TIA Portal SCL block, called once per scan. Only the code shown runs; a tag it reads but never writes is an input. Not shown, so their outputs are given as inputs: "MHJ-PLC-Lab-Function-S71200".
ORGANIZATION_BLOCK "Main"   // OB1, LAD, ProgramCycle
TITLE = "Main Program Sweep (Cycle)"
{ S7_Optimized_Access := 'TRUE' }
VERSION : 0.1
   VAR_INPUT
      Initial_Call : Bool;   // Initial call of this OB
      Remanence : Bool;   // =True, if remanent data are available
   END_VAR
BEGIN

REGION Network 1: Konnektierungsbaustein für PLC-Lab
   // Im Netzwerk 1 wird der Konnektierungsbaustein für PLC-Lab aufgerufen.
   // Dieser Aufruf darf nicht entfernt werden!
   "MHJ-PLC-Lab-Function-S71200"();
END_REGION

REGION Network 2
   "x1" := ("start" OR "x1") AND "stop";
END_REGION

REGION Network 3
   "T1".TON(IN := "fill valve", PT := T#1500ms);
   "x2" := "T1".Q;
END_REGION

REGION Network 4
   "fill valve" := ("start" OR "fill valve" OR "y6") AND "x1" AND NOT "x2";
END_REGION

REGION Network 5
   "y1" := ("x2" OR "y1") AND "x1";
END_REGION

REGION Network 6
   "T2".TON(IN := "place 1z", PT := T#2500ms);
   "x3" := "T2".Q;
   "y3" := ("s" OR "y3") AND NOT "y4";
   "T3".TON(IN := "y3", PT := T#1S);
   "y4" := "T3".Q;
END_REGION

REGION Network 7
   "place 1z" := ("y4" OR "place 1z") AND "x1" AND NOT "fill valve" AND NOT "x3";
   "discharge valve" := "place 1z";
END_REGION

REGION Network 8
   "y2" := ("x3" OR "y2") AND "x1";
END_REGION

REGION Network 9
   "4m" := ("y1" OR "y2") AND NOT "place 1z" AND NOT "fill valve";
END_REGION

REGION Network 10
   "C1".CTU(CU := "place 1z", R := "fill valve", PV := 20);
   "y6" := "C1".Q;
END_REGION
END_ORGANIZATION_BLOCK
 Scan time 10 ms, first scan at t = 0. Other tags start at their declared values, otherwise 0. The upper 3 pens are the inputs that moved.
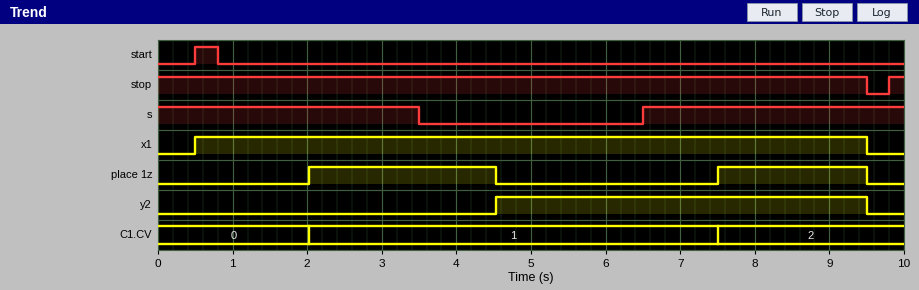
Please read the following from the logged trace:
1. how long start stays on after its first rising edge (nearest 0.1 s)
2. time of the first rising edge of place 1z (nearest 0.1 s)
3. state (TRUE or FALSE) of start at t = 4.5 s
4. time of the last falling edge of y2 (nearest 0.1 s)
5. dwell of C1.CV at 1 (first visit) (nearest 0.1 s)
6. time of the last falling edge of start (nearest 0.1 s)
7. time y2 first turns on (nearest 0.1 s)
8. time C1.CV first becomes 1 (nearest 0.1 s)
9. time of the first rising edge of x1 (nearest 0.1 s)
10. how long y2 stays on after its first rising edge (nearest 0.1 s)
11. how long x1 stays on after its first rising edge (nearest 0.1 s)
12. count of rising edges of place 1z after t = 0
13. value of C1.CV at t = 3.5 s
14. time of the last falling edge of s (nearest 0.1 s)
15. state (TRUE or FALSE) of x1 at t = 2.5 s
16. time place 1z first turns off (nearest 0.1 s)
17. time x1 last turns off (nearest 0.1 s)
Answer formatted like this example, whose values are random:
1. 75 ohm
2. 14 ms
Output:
1. 0.3 s
2. 2.0 s
3. FALSE
4. 9.5 s
5. 5.5 s
6. 0.8 s
7. 4.5 s
8. 2.0 s
9. 0.5 s
10. 5.0 s
11. 9.0 s
12. 2
13. 1
14. 3.5 s
15. TRUE
16. 4.5 s
17. 9.5 s
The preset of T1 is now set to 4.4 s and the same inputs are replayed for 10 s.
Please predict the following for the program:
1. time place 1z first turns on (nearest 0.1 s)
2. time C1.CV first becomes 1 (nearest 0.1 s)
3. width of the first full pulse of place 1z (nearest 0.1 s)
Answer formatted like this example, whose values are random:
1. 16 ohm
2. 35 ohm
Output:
1. 7.5 s
2. 7.5 s
3. 2.0 s
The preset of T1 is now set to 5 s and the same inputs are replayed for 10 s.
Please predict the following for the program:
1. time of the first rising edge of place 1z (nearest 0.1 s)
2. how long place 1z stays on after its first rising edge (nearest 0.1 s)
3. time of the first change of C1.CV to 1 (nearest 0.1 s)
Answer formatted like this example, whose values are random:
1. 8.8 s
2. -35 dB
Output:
1. 7.5 s
2. 2.0 s
3. 7.5 s
